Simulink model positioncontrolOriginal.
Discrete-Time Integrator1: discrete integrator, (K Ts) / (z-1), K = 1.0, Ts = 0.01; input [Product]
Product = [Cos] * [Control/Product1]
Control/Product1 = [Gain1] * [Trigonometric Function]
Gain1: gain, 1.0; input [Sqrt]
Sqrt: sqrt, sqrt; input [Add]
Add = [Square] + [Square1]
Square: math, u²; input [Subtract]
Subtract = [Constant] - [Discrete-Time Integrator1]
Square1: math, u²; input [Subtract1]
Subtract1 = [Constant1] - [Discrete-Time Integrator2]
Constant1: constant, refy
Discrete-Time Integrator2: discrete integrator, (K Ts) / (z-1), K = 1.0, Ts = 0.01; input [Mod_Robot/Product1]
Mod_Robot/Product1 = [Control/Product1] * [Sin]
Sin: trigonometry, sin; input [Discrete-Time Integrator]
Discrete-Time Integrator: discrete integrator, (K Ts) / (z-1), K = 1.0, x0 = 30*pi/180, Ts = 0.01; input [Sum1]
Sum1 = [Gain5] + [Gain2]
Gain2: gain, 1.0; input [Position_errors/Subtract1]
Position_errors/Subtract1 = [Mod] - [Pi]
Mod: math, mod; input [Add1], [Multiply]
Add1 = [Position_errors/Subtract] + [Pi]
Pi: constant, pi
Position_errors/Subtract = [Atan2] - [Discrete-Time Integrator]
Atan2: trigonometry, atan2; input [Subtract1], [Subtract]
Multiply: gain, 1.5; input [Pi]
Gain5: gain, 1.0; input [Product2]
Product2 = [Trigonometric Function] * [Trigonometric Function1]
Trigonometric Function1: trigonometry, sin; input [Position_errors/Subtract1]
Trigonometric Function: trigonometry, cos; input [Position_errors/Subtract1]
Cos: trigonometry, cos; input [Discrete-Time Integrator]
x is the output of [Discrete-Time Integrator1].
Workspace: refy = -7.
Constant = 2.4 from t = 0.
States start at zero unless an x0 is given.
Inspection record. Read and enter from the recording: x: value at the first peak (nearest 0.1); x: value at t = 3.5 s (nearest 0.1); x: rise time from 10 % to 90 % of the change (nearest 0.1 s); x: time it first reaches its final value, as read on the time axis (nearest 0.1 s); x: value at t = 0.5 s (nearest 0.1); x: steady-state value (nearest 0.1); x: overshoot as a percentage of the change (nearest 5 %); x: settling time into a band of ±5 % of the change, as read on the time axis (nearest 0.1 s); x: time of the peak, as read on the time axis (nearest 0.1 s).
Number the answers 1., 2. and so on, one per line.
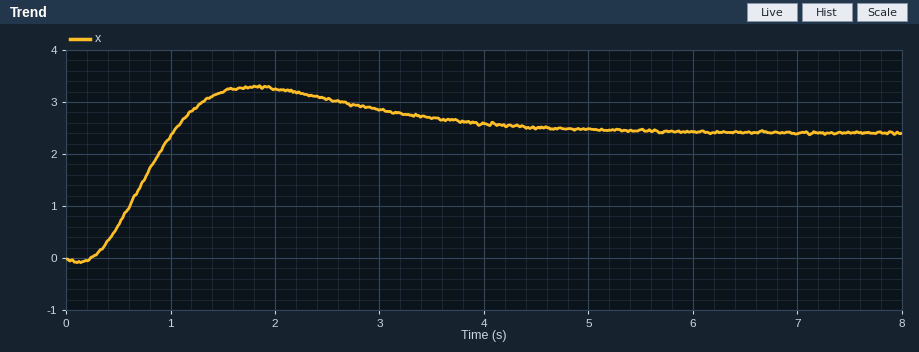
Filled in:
1. 3.3
2. 2.7
3. 0.6 s
4. 1.0 s
5. 0.6
6. 2.4
7. 35 %
8. 4.4 s
9. 1.8 s
